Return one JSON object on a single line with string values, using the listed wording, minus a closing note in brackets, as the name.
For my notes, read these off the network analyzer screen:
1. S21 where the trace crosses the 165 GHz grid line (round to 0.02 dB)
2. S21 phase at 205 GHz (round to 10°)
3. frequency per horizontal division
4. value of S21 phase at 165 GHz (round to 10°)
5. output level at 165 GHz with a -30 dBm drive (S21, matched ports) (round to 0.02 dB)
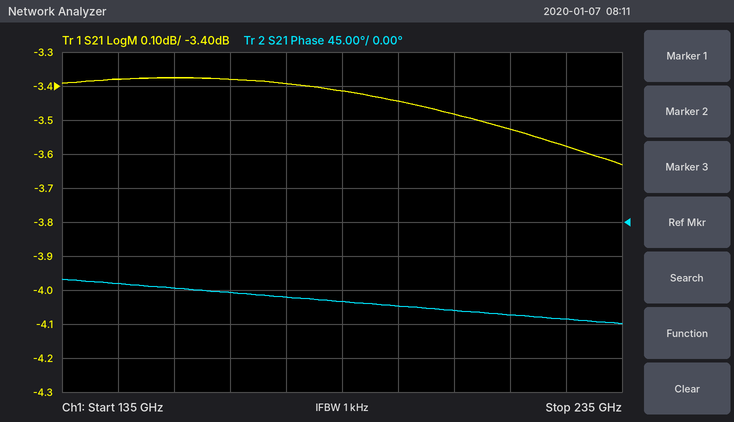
{"S21 where the trace crosses the 165 GHz grid line": "-3.38 dB", "S21 phase at 205 GHz": "-120°", "frequency per horizontal division": "10 GHz", "value of S21 phase at 165 GHz": "-90°", "output level at 165 GHz with a -30 dBm drive (S21, matched ports)": "-33.38 dBm"}
